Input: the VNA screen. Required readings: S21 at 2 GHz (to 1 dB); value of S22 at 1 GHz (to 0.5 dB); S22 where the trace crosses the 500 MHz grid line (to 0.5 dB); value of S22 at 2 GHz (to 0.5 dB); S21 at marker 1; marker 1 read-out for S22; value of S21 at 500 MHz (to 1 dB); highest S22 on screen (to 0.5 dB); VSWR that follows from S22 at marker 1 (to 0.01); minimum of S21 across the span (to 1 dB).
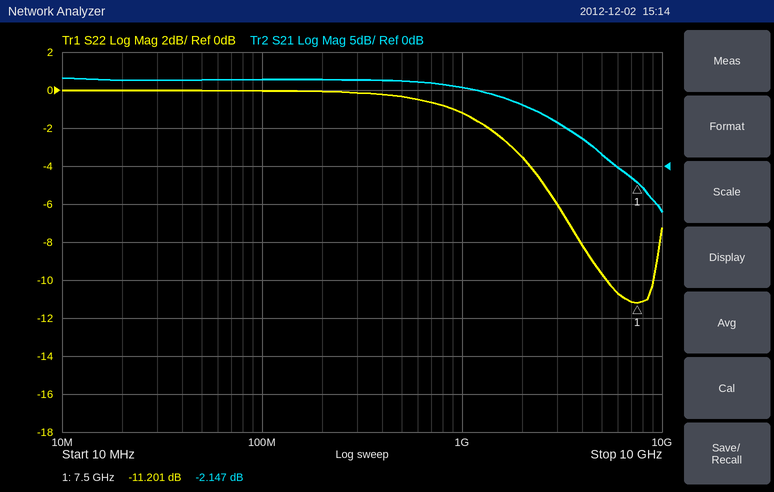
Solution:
8 dB
-1.0 dB
-0.5 dB
-3.5 dB
-2.147 dB
-11.201 dB
11 dB
0.0 dB
1.76
-6 dB
